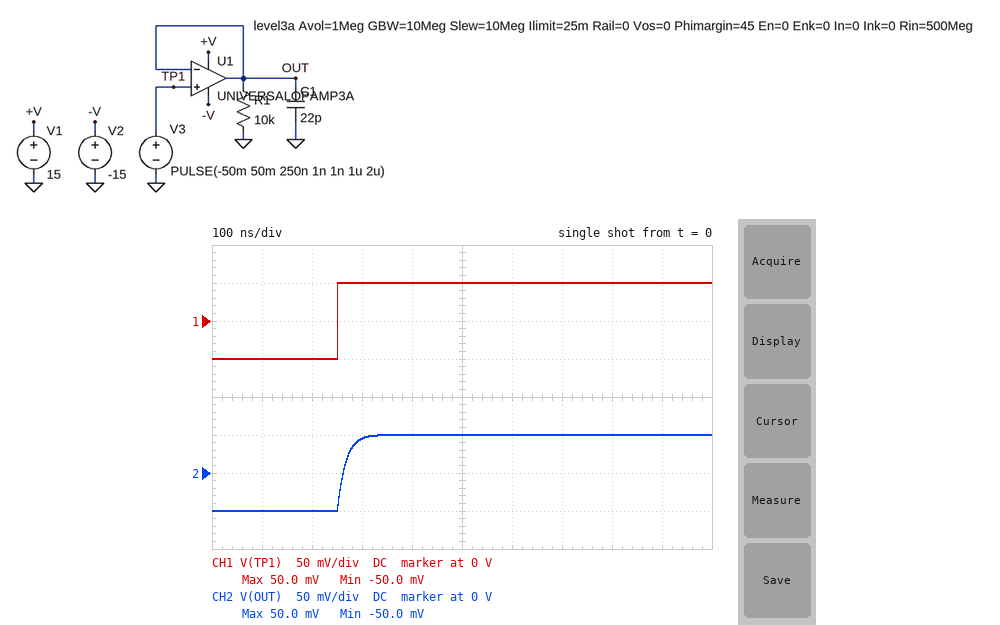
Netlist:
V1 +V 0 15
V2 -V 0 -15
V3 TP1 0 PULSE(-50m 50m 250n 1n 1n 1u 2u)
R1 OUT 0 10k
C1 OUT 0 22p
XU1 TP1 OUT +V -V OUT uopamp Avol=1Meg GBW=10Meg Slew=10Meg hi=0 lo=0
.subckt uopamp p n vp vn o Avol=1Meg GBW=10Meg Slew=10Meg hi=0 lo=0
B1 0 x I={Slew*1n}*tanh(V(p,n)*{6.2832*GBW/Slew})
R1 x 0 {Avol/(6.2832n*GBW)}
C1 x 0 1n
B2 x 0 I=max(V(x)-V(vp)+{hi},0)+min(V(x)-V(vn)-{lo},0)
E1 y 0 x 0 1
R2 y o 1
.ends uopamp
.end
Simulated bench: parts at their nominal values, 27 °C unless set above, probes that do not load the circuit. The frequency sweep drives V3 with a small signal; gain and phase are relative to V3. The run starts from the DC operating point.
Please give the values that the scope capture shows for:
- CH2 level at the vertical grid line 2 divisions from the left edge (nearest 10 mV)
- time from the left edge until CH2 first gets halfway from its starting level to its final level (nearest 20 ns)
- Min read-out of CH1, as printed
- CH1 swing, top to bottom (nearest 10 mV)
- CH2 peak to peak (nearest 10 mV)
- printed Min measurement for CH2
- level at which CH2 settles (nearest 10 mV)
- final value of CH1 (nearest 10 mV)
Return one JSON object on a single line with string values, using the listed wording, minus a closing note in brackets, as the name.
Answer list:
{"CH2 level at the vertical grid line 2 divisions from the left edge": "-50 mV", "time from the left edge until CH2 first gets halfway from its starting level to its final level": "260 ns", "Min read-out of CH1, as printed": "-50.0 mV", "CH1 swing, top to bottom": "100 mV", "CH2 peak to peak": "100 mV", "printed Min measurement for CH2": "-50.0 mV", "level at which CH2 settles": "50 mV", "final value of CH1": "50 mV"}
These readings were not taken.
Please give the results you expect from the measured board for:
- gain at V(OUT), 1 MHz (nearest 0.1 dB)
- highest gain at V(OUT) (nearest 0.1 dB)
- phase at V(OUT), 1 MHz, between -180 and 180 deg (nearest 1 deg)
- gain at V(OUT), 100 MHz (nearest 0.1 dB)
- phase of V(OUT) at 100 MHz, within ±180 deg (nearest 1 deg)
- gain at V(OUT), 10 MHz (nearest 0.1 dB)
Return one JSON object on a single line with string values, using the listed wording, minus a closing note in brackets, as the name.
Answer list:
{"gain at V(OUT), 1 MHz": "0 dB", "highest gain at V(OUT)": "0 dB", "phase at V(OUT), 1 MHz, between -180 and 180 deg": "-6 deg", "gain at V(OUT), 100 MHz": "-20.0 dB", "phase of V(OUT) at 100 MHz, within ±180 deg": "-85 deg", "gain at V(OUT), 10 MHz": "-3.0 dB"}
